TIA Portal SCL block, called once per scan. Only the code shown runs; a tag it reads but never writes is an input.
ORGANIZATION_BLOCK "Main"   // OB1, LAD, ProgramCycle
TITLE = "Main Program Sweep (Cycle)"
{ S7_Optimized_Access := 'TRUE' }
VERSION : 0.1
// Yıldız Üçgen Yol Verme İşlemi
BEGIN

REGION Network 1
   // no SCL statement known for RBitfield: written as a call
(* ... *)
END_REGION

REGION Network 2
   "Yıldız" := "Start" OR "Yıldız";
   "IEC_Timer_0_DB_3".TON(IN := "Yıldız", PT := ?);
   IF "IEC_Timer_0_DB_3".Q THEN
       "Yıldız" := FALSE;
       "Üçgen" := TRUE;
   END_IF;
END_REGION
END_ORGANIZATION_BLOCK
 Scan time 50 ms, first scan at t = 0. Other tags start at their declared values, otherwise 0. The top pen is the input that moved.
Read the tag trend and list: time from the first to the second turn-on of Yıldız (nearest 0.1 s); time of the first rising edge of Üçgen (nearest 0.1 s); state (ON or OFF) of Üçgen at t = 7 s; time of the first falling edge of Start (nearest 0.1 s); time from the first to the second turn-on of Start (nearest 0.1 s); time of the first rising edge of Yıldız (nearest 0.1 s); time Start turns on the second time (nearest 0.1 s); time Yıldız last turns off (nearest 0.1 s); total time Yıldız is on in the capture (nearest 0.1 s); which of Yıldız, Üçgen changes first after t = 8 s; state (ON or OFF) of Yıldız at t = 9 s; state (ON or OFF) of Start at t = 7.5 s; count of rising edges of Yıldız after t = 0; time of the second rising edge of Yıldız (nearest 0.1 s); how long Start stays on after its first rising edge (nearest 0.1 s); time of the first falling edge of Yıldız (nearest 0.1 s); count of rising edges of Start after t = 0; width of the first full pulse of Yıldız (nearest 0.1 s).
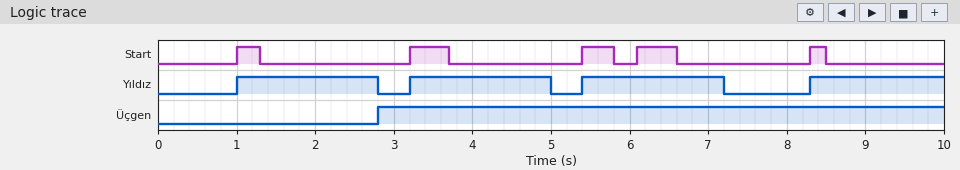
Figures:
2.2 s
2.8 s
ON
1.3 s
2.2 s
1.0 s
3.2 s
7.2 s
7.1 s
Yıldız
ON
OFF
4
3.2 s
0.3 s
2.8 s
5
1.8 s
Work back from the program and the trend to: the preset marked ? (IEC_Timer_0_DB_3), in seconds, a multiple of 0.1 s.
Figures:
1.8 s
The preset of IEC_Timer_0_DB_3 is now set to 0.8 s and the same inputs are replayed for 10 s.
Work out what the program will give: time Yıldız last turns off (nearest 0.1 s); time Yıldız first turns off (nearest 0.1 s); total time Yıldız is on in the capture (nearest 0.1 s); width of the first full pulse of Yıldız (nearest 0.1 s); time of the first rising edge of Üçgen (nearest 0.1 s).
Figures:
9.1 s
1.8 s
3.2 s
0.8 s
1.8 s
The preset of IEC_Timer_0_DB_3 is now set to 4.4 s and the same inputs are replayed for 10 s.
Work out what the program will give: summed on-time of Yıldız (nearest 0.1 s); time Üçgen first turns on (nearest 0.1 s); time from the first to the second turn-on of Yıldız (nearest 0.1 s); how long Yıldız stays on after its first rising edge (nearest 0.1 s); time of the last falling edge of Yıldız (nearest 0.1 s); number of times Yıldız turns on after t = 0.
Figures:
8.3 s
5.4 s
5.1 s
4.4 s
5.4 s
2
